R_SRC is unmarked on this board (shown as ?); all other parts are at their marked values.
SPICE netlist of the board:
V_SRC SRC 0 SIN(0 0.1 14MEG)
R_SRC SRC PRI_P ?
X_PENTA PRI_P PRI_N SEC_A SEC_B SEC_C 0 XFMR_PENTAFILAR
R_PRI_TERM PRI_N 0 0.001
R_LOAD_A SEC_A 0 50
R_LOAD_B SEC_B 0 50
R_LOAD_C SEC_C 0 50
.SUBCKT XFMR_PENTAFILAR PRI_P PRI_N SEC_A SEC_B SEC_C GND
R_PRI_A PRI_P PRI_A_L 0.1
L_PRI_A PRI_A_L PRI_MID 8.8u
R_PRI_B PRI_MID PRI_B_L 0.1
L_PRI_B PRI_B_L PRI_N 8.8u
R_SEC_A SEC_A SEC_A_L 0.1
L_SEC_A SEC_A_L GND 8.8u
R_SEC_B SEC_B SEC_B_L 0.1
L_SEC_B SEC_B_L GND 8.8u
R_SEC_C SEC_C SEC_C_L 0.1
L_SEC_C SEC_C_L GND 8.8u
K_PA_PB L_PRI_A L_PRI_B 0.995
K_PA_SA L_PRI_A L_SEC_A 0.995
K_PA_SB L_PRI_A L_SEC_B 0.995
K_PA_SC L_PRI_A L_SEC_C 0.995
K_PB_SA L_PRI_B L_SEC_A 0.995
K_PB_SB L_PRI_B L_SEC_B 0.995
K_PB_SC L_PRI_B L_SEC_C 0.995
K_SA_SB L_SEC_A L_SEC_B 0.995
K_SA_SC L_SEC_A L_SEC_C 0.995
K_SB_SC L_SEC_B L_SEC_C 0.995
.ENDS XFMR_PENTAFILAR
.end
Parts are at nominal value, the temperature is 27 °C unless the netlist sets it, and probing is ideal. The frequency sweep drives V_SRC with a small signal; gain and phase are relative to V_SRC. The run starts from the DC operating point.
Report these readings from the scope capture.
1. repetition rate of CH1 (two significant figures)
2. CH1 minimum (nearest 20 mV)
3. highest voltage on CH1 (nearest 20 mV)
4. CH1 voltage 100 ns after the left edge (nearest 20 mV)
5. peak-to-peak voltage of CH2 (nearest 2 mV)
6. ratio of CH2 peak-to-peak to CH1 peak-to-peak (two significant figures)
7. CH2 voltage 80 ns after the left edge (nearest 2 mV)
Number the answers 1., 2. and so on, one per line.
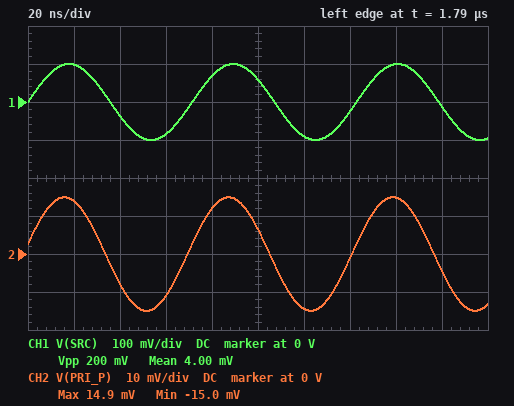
1. 14 MHz
2. -100 mV
3. 100 mV
4. 60 mV
5. 30 mV
6. 0.15
7. 12 mV
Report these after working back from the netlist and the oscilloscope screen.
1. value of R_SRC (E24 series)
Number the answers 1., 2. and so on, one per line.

1. 390 Ω
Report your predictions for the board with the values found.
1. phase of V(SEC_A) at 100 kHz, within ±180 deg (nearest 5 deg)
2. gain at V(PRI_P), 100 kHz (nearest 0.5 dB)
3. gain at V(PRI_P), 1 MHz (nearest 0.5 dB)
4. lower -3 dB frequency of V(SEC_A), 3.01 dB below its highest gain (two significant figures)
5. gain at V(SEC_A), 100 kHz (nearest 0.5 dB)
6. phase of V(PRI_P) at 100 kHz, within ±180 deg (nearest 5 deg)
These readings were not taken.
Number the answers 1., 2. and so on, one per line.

1. 70 deg
2. -25.5 dB
3. -17.0 dB
4. 260 kHz
5. -31.5 dB
6. 70 deg
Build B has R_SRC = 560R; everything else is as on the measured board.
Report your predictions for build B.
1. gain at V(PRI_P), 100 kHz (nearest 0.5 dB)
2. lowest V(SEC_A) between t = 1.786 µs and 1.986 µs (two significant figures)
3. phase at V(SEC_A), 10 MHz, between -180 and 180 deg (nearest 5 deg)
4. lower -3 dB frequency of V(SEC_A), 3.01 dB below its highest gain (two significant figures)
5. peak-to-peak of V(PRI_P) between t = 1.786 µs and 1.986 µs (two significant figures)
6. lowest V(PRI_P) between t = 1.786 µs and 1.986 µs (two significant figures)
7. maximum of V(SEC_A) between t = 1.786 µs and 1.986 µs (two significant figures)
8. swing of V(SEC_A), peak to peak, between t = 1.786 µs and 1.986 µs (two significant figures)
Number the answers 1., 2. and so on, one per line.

1. -28.5 dB
2. -5.3 mV
3. 0 deg
4. 270 kHz
5. 22 mV
6. -11 mV
7. 5.3 mV
8. 11 mV
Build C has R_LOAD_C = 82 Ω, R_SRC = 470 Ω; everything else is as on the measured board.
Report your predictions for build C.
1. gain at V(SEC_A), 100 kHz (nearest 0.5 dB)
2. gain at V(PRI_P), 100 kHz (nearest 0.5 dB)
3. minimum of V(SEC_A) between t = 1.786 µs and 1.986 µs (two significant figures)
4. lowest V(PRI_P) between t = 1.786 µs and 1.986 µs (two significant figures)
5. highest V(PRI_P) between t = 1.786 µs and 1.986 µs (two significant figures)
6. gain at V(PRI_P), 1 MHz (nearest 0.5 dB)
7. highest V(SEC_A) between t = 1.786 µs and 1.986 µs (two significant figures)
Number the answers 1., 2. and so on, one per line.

1. -33.0 dB
2. -27.0 dB
3. -7.0 mV
4. -14 mV
5. 14 mV
6. -17.5 dB
7. 7.0 mV
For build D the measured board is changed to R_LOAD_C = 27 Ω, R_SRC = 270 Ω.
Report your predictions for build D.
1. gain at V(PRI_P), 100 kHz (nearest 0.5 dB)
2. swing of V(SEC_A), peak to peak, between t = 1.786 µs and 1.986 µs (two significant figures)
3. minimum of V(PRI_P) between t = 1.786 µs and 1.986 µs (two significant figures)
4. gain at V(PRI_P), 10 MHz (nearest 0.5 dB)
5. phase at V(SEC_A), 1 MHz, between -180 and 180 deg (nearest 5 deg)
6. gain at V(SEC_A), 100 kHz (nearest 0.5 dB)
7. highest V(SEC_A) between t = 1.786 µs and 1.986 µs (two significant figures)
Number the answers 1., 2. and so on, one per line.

1. -22.5 dB
2. 16 mV
3. -17 mV
4. -15.5 dB
5. 10 deg
6. -29.0 dB
7. 8.1 mV
